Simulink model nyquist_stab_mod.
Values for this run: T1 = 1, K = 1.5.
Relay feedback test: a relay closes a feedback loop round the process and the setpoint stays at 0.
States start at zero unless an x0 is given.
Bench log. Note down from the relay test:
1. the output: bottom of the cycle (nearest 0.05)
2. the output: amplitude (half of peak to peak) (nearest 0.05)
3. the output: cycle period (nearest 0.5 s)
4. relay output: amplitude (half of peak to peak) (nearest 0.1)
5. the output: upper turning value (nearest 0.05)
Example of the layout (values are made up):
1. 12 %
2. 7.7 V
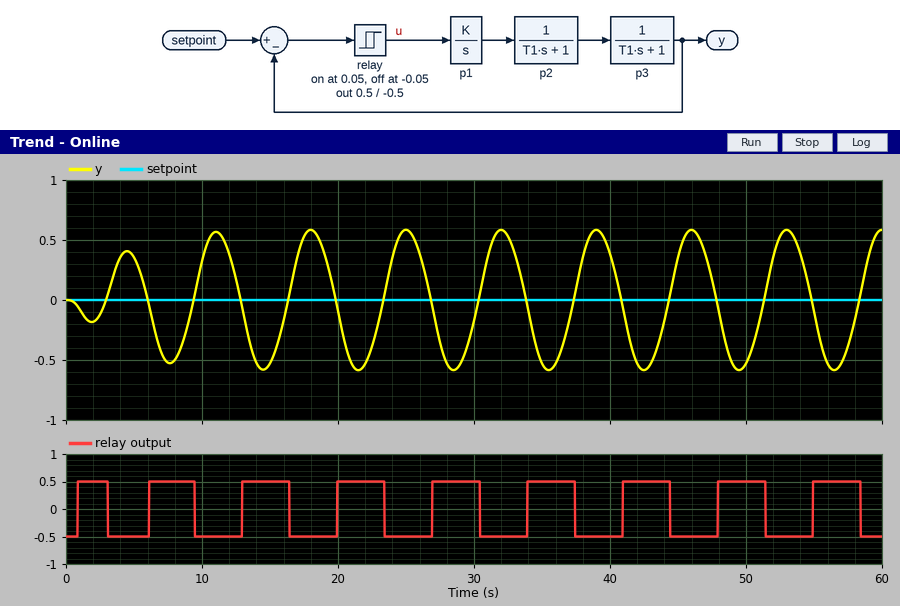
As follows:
1. -0.60
2. 0.60
3. 7.0 s
4. 0.5
5. 0.60
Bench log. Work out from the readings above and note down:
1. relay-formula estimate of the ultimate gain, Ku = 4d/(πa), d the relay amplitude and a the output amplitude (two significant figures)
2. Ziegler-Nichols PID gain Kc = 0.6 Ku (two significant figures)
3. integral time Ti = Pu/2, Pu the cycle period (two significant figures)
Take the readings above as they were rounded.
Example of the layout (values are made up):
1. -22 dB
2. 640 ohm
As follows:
1. 1.1
2. 0.66
3. 3.5 s
